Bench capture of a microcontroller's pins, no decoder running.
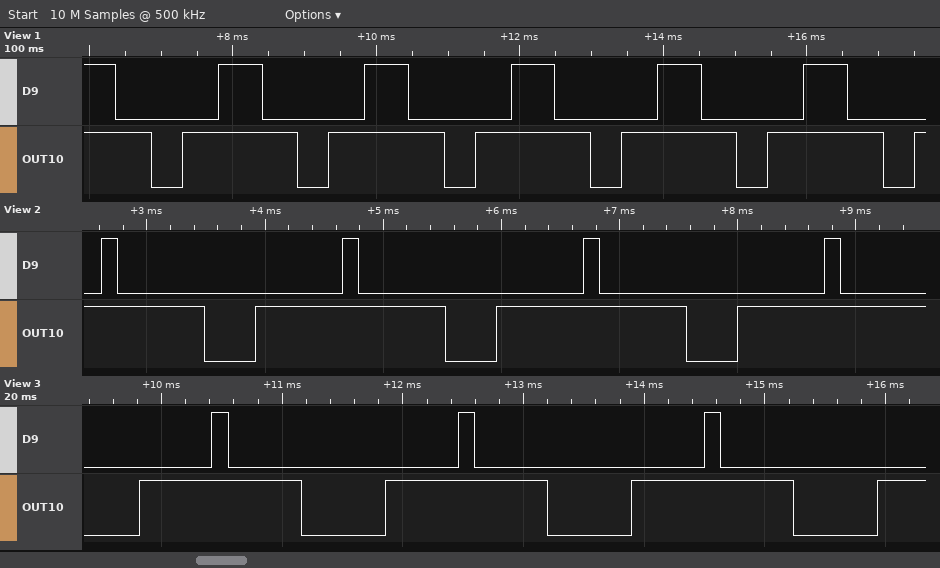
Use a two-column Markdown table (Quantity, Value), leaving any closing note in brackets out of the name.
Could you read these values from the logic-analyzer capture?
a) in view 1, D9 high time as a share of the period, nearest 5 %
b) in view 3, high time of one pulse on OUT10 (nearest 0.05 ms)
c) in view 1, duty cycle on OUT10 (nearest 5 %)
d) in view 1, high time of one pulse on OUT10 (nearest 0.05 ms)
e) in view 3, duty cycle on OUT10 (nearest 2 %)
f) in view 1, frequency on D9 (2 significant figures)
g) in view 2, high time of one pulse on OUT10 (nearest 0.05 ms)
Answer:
| Quantity | Value |
|---|---|
| in view 1, D9 high time as a share of the period, nearest 5 % | 30 % |
| in view 3, high time of one pulse on OUT10 | 1.35 ms |
| in view 1, duty cycle on OUT10 | 80 % |
| in view 1, high time of one pulse on OUT10 | 1.60 ms |
| in view 3, duty cycle on OUT10 | 66 % |
| in view 1, frequency on D9 | 490 Hz |
| in view 2, high time of one pulse on OUT10 | 1.60 ms |
